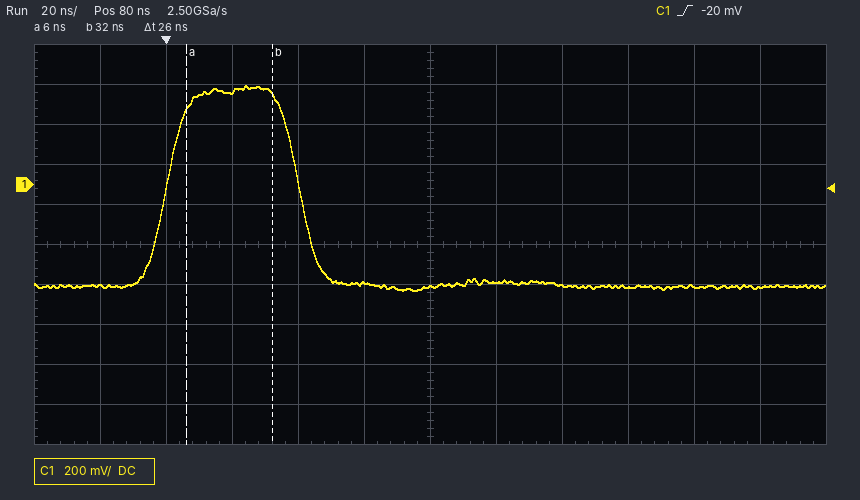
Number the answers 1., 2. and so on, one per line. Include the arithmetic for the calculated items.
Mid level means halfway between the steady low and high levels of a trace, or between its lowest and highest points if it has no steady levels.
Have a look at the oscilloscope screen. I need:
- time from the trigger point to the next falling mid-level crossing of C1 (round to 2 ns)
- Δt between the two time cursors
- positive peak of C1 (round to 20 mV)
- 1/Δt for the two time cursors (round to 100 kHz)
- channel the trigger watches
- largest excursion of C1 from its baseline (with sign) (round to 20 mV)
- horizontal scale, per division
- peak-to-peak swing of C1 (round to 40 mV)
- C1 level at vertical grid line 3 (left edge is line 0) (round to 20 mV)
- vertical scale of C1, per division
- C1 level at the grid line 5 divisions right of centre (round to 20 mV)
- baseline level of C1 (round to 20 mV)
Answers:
1. 40 ns
2. 26 ns
3. 500 mV
4. 1 / 26 ns ≈ 38.5 MHz
5. C1
6. 500 mV − (-500 mV) = +1.00 V
7. 20 ns
8. 1.04 V
9. 460 mV
10. 200 mV
11. -520 mV
12. -500 mV
